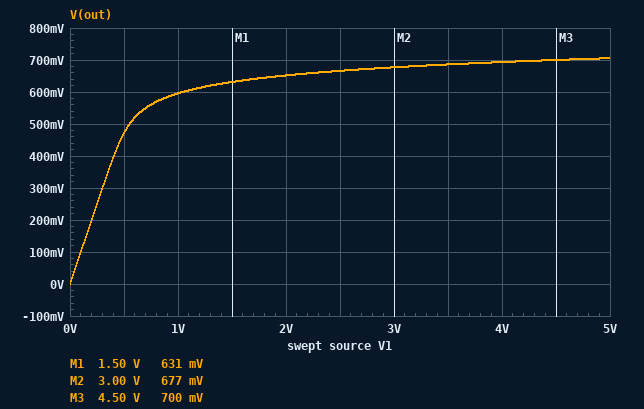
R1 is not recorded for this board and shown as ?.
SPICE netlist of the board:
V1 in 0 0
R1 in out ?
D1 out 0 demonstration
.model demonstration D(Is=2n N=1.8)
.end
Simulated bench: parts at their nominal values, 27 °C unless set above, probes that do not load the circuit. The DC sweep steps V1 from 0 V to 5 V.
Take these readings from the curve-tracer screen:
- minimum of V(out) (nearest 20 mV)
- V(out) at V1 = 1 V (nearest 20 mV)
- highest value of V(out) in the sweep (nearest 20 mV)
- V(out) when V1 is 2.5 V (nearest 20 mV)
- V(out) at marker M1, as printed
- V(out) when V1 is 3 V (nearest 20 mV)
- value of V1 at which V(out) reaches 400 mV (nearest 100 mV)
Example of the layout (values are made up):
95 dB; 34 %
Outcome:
0 V; 600 mV; 700 mV; 660 mV; 631 mV; 680 mV; 400 mV
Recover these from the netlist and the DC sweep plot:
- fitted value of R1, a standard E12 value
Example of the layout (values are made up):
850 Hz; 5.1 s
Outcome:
560 Ω
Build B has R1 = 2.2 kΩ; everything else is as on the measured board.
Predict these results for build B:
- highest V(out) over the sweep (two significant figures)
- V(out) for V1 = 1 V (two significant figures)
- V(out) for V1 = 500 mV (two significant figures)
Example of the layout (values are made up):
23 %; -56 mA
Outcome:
640 mV; 540 mV; 440 mV
